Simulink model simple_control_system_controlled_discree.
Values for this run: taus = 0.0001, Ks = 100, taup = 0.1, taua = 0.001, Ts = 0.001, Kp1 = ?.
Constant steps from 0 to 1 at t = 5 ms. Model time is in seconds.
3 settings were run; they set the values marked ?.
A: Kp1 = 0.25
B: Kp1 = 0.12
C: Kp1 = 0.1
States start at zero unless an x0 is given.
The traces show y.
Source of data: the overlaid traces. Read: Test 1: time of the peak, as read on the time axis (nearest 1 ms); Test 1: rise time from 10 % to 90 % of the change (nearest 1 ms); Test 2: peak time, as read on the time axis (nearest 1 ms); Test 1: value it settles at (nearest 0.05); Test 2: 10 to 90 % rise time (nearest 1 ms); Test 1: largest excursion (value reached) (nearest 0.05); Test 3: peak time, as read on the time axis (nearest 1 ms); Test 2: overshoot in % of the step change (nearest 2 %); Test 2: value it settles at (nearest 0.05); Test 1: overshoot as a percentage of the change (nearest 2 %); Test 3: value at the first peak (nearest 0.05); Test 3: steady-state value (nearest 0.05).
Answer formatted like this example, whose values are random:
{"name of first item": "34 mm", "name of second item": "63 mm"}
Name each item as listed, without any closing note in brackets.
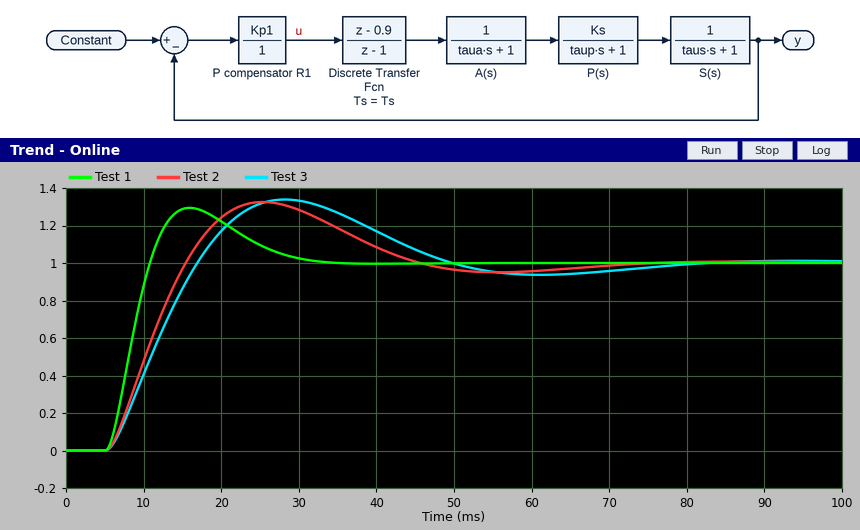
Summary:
{"Test 1: time of the peak, as read on the time axis": "16 ms", "Test 1: rise time from 10 % to 90 % of the change": "4 ms", "Test 2: peak time, as read on the time axis": "25 ms", "Test 1: value it settles at": "1.00", "Test 2: 10 to 90 % rise time": "7 ms", "Test 1: largest excursion (value reached)": "1.30", "Test 3: peak time, as read on the time axis": "28 ms", "Test 2: overshoot in % of the step change": "32 %", "Test 2: value it settles at": "1.00", "Test 1: overshoot as a percentage of the change": "30 %", "Test 3: value at the first peak": "1.35", "Test 3: steady-state value": "1.00"}
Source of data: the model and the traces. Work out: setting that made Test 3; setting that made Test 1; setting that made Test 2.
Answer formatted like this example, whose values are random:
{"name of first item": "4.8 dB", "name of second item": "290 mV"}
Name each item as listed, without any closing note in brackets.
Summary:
{"setting that made Test 3": "C", "setting that made Test 1": "A", "setting that made Test 2": "B"}
